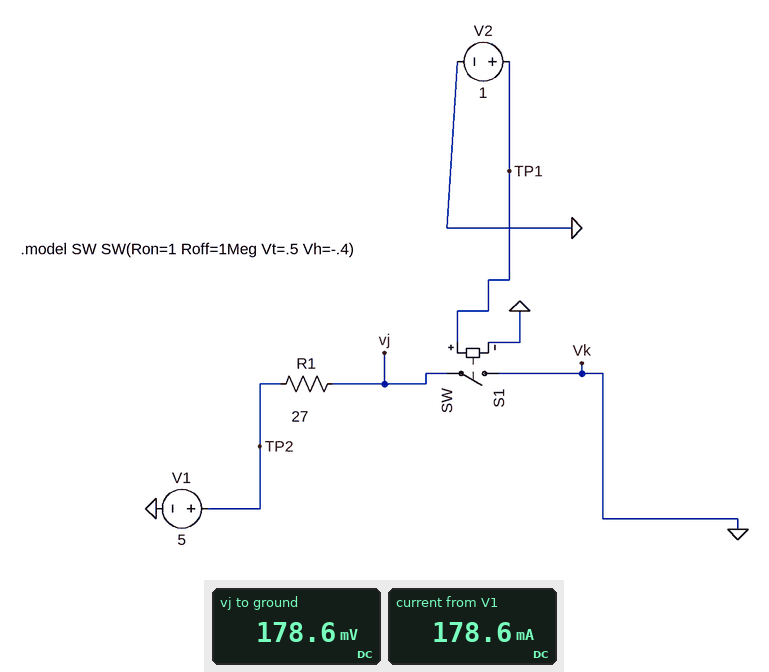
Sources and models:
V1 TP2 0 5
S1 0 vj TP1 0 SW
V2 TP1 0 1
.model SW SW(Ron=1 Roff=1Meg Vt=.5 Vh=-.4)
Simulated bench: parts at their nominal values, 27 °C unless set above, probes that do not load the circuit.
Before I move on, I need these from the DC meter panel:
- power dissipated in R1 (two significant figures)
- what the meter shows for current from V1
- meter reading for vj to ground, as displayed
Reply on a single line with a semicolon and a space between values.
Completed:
860 mW; 178.6 mA; 178.6 mV
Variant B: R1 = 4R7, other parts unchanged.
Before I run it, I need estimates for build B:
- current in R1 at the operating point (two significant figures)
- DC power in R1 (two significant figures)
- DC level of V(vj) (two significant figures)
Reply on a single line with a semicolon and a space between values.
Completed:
880 mA; 3.6 W; 880 mV
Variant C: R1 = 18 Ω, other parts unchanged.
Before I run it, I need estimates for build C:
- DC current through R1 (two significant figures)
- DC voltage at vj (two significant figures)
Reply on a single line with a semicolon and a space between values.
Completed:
260 mA; 260 mV
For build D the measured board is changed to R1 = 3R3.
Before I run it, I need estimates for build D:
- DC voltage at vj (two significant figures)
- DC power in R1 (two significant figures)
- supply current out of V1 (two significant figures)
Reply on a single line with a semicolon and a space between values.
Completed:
1.2 V; 4.5 W; 1.2 A
